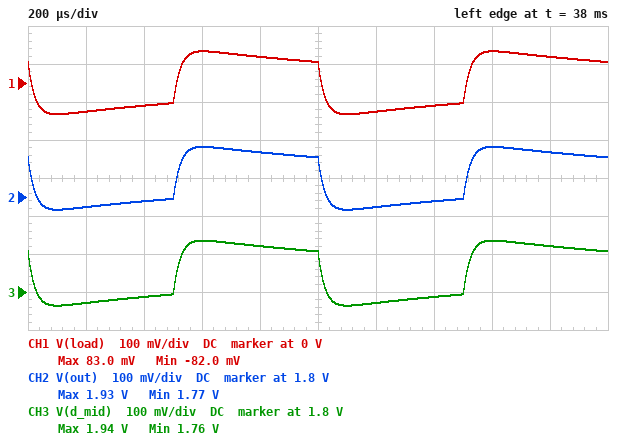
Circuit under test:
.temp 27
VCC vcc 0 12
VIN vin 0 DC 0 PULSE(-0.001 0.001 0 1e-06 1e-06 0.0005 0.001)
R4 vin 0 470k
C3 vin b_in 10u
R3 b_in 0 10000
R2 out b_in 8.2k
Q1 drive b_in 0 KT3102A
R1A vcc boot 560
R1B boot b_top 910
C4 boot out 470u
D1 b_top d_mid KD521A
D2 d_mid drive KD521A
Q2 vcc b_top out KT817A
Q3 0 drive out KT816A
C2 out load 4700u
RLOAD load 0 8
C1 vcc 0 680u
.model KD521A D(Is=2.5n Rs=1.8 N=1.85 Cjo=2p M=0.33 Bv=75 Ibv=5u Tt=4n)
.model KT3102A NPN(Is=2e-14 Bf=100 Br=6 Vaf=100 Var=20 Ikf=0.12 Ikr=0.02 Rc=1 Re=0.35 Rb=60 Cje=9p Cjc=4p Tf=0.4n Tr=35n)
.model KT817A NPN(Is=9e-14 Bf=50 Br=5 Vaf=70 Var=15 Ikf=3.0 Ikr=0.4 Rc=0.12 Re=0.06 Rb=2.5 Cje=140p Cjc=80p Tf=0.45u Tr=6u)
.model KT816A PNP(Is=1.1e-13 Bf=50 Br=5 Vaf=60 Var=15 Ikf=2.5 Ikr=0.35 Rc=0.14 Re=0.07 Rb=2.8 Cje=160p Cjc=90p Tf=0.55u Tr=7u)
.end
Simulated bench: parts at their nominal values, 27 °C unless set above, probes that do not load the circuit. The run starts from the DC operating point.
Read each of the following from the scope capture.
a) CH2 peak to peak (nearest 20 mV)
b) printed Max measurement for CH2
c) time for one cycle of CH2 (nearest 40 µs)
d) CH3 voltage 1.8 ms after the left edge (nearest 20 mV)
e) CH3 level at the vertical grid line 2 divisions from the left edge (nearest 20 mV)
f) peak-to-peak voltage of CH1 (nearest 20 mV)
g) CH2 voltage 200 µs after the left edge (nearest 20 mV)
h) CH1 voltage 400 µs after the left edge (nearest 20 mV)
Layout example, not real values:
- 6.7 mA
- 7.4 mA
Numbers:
- 160 mV
- 1.93 V
- 1.00 ms
- 1.92 V
- 1.78 V
- 160 mV
- 1.78 V
- -60 mV
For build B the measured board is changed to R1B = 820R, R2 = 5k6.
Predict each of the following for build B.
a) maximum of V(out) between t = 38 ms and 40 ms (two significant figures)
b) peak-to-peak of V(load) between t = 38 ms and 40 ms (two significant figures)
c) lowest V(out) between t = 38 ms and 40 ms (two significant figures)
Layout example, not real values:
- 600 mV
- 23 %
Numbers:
- 1.6 V
- 190 mV
- 1.4 V
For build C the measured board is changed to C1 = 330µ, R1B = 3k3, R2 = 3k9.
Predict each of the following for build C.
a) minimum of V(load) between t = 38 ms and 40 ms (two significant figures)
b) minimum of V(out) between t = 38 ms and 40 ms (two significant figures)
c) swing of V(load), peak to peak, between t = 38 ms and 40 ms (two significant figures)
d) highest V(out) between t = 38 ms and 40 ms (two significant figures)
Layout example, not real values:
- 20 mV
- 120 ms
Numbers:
- -42 mV
- 1.0 V
- 84 mV
- 1.1 V
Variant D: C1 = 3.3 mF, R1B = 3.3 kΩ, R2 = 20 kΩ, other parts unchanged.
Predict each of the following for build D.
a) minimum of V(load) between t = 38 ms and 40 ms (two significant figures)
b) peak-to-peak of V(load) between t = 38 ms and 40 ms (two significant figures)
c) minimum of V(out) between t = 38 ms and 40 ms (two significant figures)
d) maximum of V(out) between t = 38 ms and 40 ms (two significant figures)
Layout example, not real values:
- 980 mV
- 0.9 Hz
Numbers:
- -32 mV
- 66 mV
- 2.4 V
- 2.5 V
